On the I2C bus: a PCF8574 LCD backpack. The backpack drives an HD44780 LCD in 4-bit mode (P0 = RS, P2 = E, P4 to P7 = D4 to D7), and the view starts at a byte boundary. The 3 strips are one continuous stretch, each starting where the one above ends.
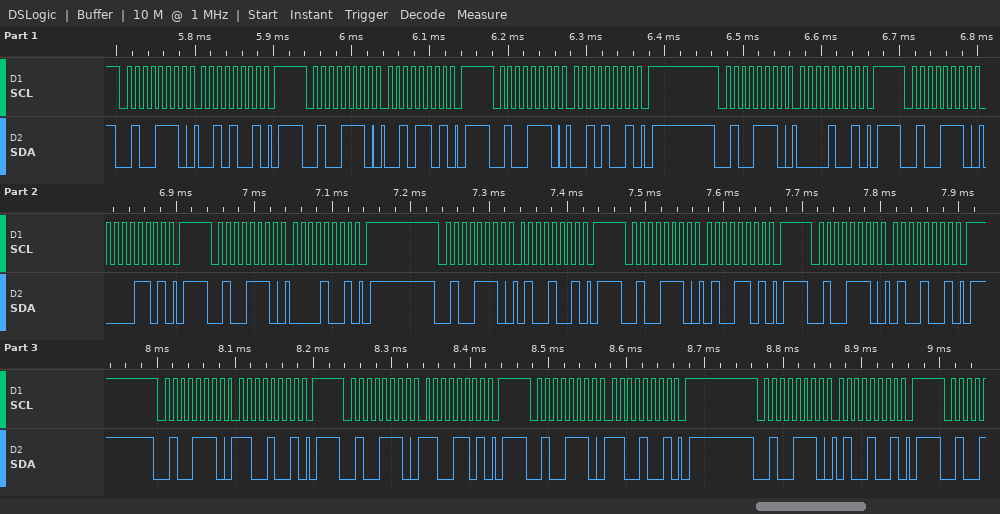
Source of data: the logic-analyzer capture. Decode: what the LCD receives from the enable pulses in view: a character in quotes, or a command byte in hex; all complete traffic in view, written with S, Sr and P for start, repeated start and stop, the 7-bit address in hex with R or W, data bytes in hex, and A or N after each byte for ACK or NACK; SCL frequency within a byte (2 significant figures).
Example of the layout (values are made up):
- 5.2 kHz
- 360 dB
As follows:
- ' ' 'L'
- S 27W A 29 A P S 27W A 2D A P S 27W A 29 A P S 27W A 09 A P S 27W A 0D A P S 27W A 09 A P S 27W A 49 A P S 27W A 4D A P S 27W A 49 A P S 27W A C9 A P S 27W A CD A P S 27W A C9 A P S 27W A 49 A P
- 100 kHz
